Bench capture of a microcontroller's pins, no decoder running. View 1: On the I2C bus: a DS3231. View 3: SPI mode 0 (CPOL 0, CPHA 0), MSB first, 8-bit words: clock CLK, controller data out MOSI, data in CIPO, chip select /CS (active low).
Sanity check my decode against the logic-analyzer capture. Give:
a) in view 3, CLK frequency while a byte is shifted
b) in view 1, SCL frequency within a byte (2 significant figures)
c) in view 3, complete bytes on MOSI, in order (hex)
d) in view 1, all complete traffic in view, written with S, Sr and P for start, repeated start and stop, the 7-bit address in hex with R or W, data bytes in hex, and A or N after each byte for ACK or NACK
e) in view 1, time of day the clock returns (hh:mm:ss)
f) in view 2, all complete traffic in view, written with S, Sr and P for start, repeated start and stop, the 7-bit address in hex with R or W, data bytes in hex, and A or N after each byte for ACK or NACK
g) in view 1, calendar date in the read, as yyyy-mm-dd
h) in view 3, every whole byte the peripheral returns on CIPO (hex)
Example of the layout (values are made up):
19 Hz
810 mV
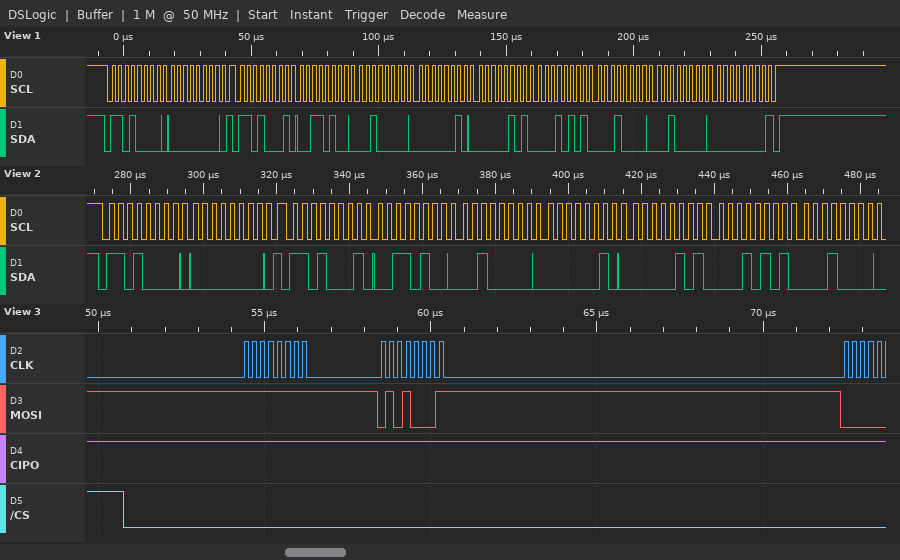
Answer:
4 MHz
400 kHz
0xFF 0x51
S 68W A 00 A Sr 68R A 34 A 20 A 02 A 05 A 15 A 10 A 20 A 00 N P
02:20:34
S 68W A 00 A Sr 68R A 34 A 20 A 02 A 05 A 15 A 10 A
2020-10-15
0xFF 0xFF
